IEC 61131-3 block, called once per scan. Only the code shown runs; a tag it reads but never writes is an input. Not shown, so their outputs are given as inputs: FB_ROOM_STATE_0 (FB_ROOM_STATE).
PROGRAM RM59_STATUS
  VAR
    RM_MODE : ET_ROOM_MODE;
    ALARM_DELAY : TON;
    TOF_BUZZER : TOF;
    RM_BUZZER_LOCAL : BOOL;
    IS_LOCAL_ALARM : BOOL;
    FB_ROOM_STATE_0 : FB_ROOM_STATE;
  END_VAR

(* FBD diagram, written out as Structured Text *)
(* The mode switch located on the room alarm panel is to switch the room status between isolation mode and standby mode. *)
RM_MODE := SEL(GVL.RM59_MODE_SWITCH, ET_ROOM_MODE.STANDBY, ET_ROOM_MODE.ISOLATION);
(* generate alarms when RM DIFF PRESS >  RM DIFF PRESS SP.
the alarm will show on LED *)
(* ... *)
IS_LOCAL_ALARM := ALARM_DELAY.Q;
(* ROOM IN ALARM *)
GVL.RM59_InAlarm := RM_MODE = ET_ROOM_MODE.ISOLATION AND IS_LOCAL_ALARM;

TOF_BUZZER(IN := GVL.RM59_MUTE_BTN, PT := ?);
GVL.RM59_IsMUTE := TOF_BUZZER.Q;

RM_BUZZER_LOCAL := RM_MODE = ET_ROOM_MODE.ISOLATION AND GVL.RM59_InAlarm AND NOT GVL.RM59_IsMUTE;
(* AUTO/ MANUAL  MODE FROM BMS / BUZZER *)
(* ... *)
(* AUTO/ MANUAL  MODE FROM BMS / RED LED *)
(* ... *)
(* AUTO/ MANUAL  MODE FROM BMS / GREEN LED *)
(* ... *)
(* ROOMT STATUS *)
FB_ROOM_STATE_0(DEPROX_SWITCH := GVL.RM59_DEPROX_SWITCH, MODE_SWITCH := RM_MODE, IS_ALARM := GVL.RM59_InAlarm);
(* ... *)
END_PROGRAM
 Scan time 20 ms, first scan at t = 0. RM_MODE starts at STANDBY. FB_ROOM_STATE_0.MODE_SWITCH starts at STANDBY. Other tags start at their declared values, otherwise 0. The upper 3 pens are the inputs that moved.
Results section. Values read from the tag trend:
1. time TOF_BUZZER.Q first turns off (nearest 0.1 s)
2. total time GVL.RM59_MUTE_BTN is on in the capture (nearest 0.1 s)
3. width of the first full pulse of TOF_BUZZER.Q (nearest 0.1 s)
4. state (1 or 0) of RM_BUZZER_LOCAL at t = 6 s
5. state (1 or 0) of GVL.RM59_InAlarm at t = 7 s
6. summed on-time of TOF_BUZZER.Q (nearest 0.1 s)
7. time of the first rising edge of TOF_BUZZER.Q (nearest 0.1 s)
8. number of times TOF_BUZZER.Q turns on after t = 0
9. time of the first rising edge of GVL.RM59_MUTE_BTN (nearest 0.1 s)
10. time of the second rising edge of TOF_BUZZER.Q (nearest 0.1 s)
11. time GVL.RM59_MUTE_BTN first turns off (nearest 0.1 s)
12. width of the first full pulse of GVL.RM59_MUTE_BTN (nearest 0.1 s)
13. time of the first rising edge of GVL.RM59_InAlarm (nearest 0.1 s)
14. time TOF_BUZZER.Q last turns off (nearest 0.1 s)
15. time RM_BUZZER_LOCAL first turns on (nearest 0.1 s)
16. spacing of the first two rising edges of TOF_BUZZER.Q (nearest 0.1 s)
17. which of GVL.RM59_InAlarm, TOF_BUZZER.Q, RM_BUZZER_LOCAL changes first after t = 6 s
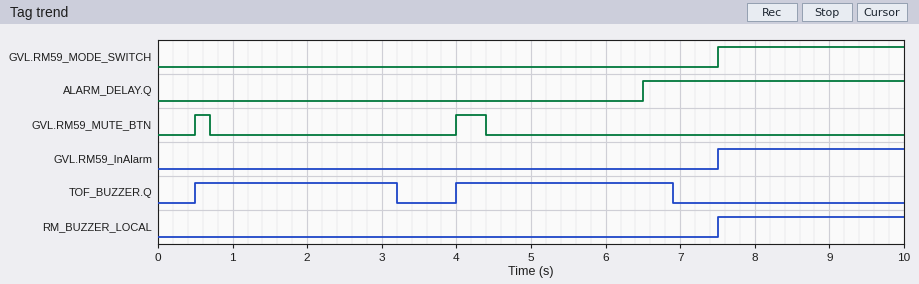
3.2 s
0.6 s
2.7 s
0
0
5.6 s
0.5 s
2
0.5 s
4.0 s
0.7 s
0.2 s
7.5 s
6.9 s
7.5 s
3.5 s
TOF_BUZZER.Q
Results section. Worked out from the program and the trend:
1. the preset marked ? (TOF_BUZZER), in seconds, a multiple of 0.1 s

2.5 s
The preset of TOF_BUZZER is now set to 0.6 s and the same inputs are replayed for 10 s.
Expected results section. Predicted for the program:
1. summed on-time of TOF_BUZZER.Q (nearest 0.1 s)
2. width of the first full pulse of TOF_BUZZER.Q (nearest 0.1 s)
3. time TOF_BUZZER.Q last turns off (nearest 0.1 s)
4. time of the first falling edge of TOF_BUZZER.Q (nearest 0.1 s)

1.8 s
0.8 s
5.0 s
1.3 s
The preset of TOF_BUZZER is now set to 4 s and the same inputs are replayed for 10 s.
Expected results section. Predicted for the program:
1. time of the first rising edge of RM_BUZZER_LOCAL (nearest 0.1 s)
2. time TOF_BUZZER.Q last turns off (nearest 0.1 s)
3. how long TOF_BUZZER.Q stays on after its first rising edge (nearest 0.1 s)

8.4 s
8.4 s
7.9 s
